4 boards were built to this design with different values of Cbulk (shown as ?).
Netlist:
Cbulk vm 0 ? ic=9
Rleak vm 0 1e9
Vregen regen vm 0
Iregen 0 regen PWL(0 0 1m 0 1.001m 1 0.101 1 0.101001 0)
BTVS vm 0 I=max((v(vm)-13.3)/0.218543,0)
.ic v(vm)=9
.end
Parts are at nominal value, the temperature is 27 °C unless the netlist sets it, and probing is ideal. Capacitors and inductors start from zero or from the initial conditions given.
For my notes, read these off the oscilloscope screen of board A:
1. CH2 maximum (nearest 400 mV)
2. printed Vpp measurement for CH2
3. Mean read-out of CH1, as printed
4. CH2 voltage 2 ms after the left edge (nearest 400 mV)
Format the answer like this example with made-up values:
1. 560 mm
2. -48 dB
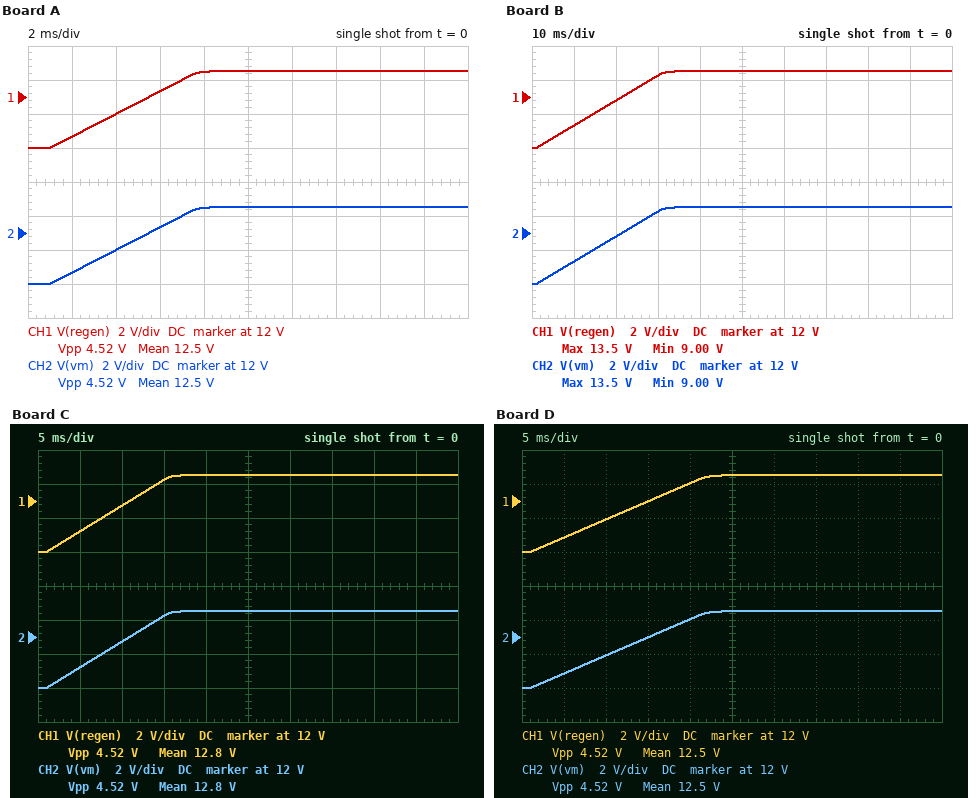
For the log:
1. 13.6 V
2. 4.52 V
3. 12.5 V
4. 9.6 V
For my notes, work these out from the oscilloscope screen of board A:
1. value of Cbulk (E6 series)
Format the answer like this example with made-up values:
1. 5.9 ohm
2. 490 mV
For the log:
1. 1.5 mF
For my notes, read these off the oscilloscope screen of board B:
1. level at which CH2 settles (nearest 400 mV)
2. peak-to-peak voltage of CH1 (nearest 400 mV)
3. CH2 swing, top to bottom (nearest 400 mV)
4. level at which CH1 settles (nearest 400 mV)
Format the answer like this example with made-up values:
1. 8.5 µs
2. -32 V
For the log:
1. 13.6 V
2. 4.4 V
3. 4.4 V
4. 13.6 V
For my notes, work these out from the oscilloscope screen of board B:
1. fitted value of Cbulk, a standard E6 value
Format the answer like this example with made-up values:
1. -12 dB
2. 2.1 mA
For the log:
1. 6.8 mF
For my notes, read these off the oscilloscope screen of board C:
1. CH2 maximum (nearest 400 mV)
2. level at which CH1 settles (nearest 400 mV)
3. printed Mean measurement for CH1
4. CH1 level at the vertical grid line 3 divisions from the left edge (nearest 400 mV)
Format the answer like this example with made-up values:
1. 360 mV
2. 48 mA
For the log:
1. 13.6 V
2. 13.6 V
3. 12.8 V
4. 13.2 V
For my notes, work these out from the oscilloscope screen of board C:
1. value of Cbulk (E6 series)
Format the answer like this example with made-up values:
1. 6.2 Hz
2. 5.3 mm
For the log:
1. 3.3 mF
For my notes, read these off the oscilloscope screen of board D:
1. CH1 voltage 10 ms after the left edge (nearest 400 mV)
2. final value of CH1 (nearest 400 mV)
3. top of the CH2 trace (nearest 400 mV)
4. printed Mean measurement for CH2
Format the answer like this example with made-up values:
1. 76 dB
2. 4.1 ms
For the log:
1. 10.8 V
2. 13.6 V
3. 13.6 V
4. 12.5 V
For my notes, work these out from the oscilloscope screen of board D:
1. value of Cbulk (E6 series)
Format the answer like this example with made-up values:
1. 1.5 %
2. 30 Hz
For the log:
1. 4.7 mF
